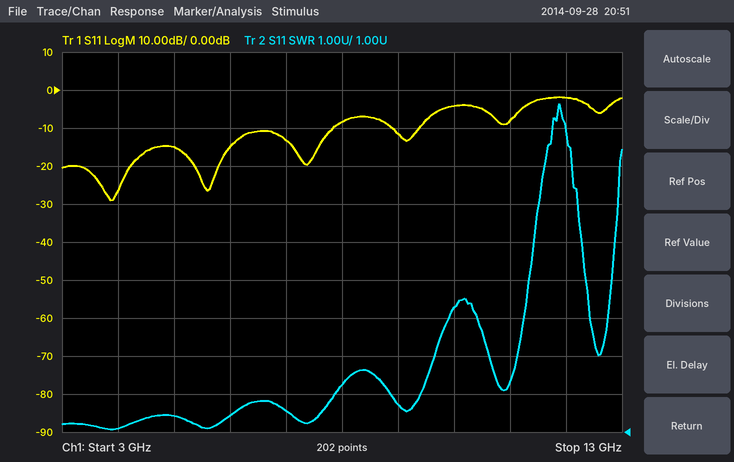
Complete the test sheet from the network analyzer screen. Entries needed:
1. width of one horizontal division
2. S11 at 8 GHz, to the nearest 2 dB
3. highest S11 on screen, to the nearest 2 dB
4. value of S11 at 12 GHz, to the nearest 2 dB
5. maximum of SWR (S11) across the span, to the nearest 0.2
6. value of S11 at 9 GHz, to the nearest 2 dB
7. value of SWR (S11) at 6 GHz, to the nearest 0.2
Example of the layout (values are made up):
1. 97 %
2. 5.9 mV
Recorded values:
1. 1 GHz
2. -8 dB
3. -2 dB
4. -2 dB
5. 9.6
6. -12 dB
7. 1.4
